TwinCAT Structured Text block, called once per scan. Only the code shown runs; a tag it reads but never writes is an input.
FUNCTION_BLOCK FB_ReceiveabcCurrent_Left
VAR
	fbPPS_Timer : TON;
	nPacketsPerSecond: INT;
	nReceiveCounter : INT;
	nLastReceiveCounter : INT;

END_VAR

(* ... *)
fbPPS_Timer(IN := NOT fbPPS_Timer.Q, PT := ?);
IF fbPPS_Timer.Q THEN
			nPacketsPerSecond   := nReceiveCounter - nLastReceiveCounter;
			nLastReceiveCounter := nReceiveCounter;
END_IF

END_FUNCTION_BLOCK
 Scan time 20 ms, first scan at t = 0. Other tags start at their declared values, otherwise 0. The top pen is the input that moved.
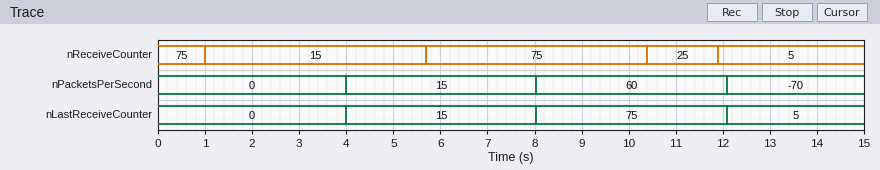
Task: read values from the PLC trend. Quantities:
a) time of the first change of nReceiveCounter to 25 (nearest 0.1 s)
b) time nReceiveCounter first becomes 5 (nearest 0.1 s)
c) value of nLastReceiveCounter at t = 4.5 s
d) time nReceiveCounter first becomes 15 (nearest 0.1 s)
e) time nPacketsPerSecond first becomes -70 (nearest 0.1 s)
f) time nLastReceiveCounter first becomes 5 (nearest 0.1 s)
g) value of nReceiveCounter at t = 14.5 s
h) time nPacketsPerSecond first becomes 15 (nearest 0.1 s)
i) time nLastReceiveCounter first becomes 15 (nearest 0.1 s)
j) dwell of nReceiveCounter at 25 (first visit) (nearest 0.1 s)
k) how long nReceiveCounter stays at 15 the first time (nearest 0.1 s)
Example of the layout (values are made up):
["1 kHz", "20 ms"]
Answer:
["10.4 s", "11.9 s", "15", "1.0 s", "12.1 s", "12.1 s", "5", "4.0 s", "4.0 s", "1.5 s", "4.7 s"]
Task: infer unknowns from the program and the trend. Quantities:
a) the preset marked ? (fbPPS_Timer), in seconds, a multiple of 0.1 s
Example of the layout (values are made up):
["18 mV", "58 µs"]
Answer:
["4.0 s"]
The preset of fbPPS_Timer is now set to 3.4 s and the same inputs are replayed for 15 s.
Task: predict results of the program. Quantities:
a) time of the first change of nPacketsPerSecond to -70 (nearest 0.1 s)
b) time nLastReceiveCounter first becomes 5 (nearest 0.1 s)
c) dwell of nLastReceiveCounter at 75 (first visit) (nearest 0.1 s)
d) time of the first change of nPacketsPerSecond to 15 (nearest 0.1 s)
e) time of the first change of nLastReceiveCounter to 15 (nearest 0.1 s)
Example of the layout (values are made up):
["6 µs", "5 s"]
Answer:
["13.7 s", "13.7 s", "6.9 s", "3.4 s", "3.4 s"]
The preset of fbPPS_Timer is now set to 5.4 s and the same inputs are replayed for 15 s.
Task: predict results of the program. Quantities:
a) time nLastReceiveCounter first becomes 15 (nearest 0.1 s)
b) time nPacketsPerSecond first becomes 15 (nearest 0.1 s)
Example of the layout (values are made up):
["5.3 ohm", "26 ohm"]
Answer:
["5.4 s", "5.4 s"]
